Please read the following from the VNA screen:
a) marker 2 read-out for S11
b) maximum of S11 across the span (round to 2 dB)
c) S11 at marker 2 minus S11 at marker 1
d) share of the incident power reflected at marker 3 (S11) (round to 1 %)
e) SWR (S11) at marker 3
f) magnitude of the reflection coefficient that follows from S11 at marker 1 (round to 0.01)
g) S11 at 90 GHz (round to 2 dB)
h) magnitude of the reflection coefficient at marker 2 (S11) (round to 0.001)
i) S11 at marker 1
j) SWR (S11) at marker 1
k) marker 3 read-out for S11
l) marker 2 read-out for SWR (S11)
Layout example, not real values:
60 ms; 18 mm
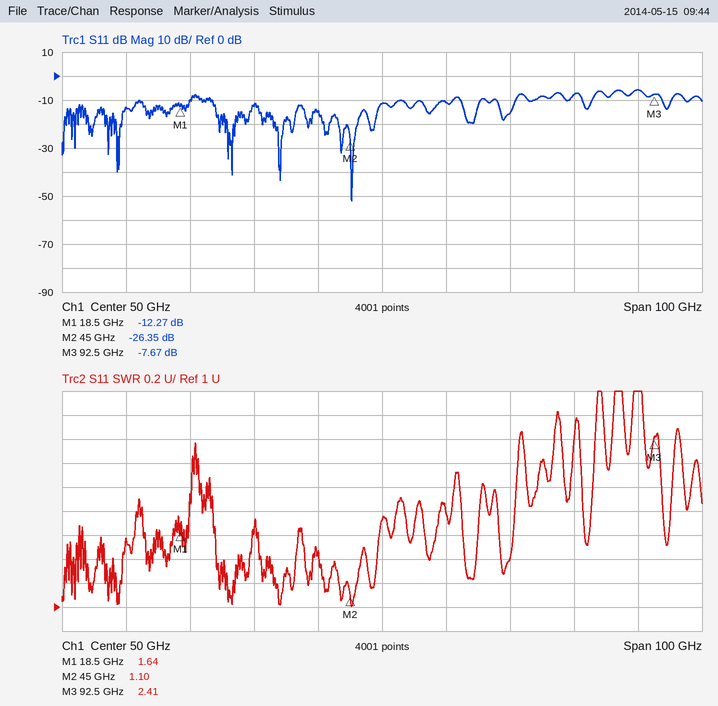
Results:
-26.35 dB; -6 dB; -14.08 dB; 17 %; 2.41; 0.24; -6 dB; 0.048; -12.27 dB; 1.64; -7.67 dB; 1.10
